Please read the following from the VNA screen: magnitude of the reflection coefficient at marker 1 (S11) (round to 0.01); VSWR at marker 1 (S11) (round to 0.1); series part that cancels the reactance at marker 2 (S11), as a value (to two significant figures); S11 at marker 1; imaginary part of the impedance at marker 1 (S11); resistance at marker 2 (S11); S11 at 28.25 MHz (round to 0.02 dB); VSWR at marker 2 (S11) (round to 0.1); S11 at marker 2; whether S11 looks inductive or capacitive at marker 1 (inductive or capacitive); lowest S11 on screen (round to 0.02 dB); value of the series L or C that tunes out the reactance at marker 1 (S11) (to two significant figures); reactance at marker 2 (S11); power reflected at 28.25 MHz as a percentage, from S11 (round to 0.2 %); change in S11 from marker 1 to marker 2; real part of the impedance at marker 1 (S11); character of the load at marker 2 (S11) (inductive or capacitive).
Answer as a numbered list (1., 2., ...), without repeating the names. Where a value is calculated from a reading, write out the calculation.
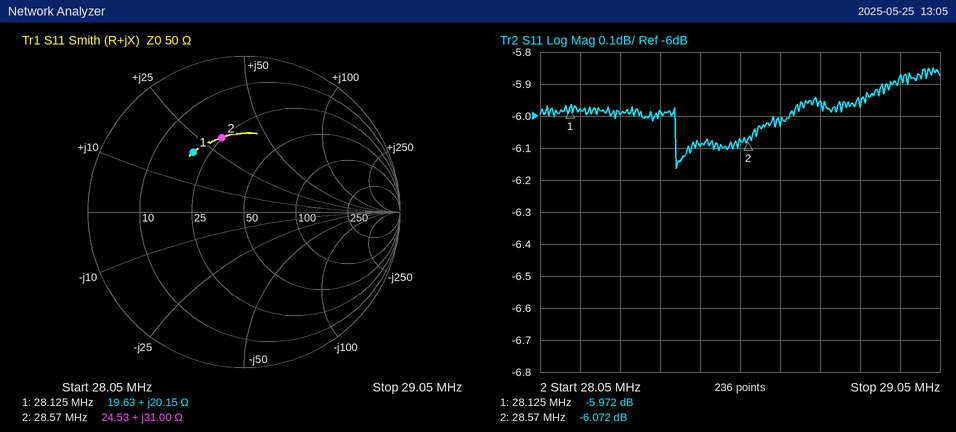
1. 0.50
2. (1 + 0.5028)/(1 − 0.5028) ≈ 3.0
3. C = 1/(2π × 28.57 MHz × 31 Ω) ≈ 180 pF
4. -5.972 dB
5. +20.15 Ω
6. 24.53 Ω
7. -6.00 dB
8. 3.0
9. -6.072 dB
10. inductive
11. -6.16 dB
12. C = 1/(2π × 28.125 MHz × 20.15 Ω) ≈ 281 pF, so 280 pF to two significant figures
13. +31.00 Ω
14. 10^(-6/10) ≈ 25.1 %, so 25.2 % to the nearest 0.2 %
15. -6.072 − (-5.972) = -0.100 dB
16. 19.63 Ω
17. inductive
